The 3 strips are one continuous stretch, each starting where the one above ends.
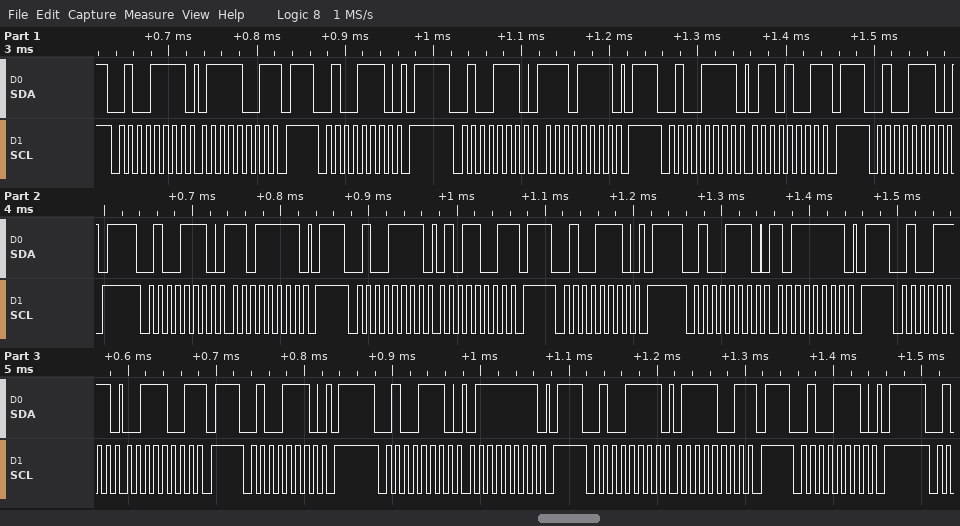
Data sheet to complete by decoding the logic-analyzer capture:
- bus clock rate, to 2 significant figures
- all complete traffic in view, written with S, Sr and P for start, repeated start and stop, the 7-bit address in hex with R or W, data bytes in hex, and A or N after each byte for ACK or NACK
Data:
100 kHz
S 27R A 79 N P S 27W A P S 27W A EF A P S 27R A 69 N P S 27W A P S 27W A DF A P S 27R A 59 N P S 27W A P S 27W A BF A P S 27R A 39 N P S 27W A P S 27W A 7F A P S 27R A 79 N P S 27W A P
